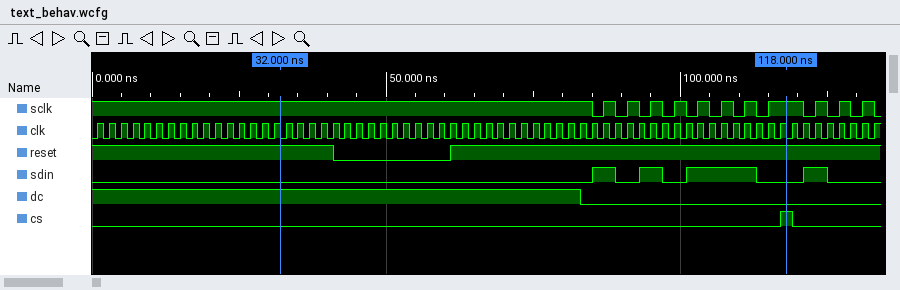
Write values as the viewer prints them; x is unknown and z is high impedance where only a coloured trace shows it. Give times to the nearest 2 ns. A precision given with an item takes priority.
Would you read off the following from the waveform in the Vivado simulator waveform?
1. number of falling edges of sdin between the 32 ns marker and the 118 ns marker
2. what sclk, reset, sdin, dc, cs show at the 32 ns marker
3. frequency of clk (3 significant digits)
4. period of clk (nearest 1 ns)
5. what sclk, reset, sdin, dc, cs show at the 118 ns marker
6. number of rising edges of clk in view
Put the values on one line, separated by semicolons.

3; sclk=1, reset=1, sdin=0, dc=1, cs=0; 500 MHz; 2 ns; sclk=1, reset=1, sdin=0, dc=0, cs=1; 67
